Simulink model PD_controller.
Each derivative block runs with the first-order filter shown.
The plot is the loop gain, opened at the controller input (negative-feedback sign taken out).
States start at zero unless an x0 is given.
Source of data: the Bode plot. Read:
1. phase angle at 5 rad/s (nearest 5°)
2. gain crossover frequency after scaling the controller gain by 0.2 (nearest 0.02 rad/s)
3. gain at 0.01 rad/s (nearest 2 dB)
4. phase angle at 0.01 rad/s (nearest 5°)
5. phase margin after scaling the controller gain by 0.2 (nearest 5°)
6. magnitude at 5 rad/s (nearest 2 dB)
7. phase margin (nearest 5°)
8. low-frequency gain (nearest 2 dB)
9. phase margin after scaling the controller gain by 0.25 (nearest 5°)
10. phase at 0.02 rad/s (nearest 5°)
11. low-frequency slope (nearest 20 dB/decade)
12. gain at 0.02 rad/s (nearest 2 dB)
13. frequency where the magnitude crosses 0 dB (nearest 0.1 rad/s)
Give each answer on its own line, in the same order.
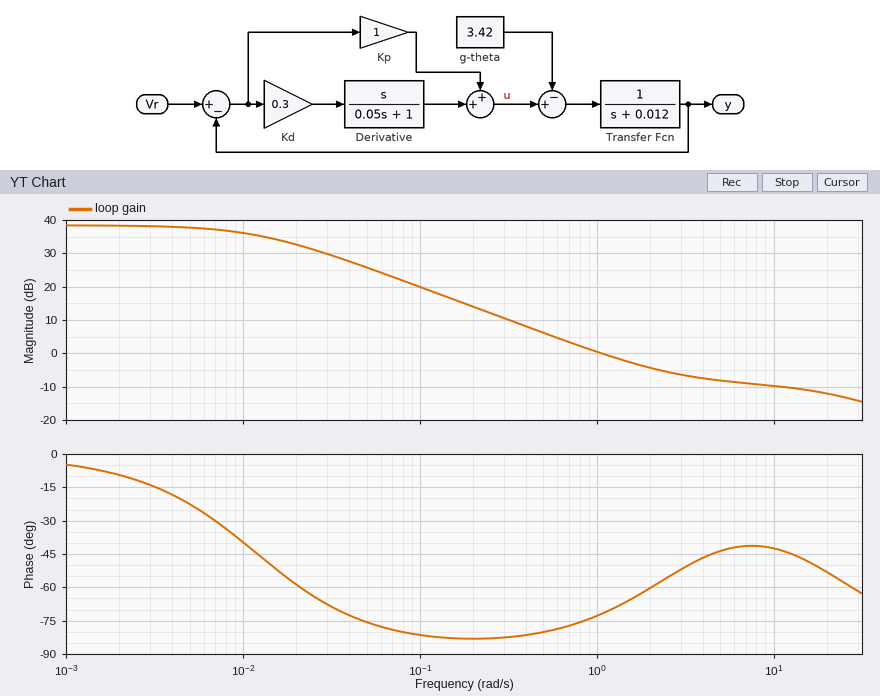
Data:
-45°
0.20 rad/s
36 dB
-40°
95°
-8 dB
110°
38 dB
95°
-60°
0 dB/decade
32 dB
1.1 rad/s
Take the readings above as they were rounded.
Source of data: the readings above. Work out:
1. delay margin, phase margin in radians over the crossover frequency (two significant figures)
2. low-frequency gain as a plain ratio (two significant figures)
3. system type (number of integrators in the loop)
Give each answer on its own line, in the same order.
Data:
1.7 s
79
0
